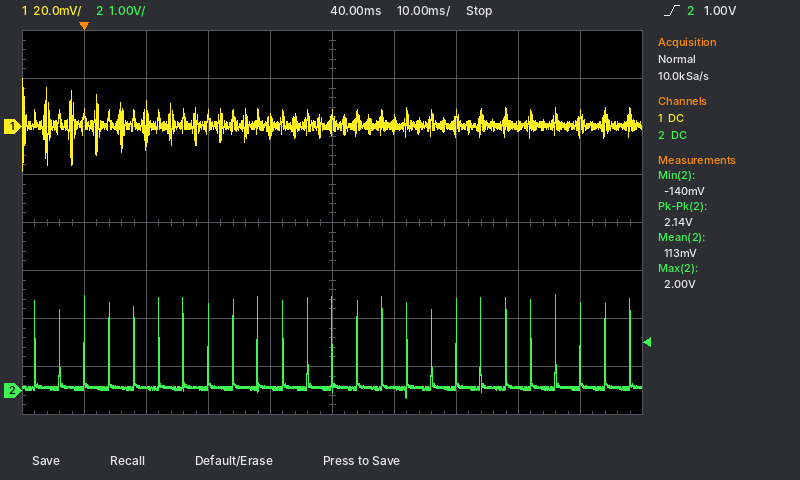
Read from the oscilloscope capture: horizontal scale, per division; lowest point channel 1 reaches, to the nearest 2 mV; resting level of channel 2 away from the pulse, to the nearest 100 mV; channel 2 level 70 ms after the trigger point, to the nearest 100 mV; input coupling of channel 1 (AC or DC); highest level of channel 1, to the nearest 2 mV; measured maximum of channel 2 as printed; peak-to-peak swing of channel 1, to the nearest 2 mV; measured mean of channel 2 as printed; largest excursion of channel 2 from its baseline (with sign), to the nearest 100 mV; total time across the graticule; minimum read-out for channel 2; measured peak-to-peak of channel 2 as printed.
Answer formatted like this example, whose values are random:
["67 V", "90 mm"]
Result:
["10 ms", "-18 mV", "100 mV", "100 mV", "DC", "20 mV", "2.00 V", "38 mV", "113 mV", "+1.9 V", "100 ms", "-140 mV", "2.14 V"]
